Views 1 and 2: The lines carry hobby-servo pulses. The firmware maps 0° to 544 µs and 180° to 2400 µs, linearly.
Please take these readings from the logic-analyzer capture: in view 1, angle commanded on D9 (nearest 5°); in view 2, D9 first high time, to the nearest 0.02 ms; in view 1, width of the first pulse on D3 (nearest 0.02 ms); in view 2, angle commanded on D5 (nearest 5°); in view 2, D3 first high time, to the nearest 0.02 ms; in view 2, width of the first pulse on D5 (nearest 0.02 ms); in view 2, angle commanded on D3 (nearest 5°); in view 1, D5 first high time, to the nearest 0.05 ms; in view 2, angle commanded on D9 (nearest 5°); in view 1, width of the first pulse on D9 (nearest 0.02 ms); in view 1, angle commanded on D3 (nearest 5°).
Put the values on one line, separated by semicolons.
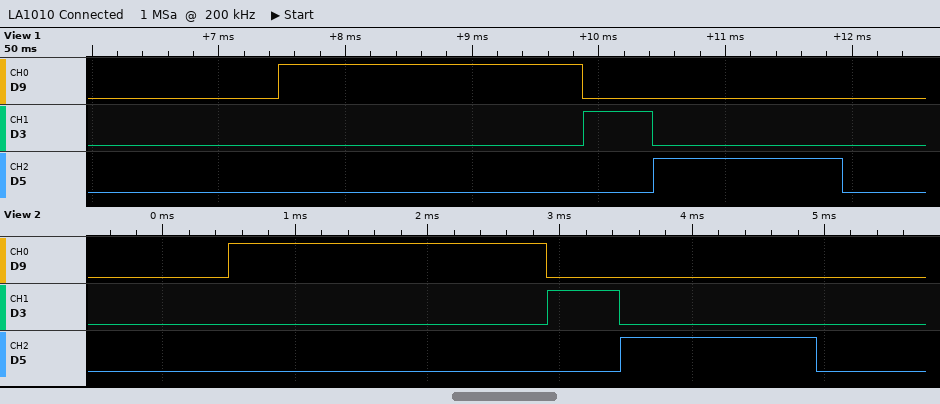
180°; 2.40 ms; 0.54 ms; 90°; 0.54 ms; 1.48 ms; 0°; 1.50 ms; 180°; 2.40 ms; 0°
